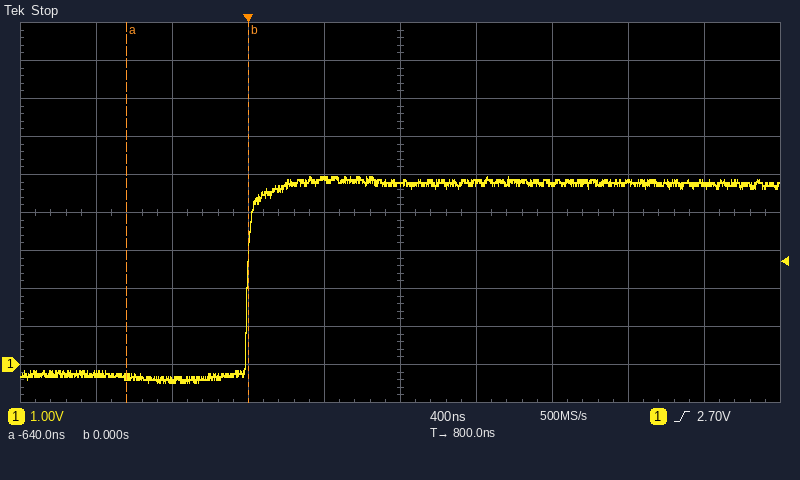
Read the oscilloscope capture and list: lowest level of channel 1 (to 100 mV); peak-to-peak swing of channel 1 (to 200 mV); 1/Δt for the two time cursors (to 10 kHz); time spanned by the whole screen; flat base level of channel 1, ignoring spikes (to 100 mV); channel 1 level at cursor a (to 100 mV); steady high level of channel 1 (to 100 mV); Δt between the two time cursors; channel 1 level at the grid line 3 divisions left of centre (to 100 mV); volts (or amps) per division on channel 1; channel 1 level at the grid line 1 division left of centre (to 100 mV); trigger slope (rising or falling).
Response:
-500 mV
5.4 V
1.56 MHz
4 µs
-300 mV
-300 mV
4.8 V
640 ns
-400 mV
1 V
4.9 V
rising
